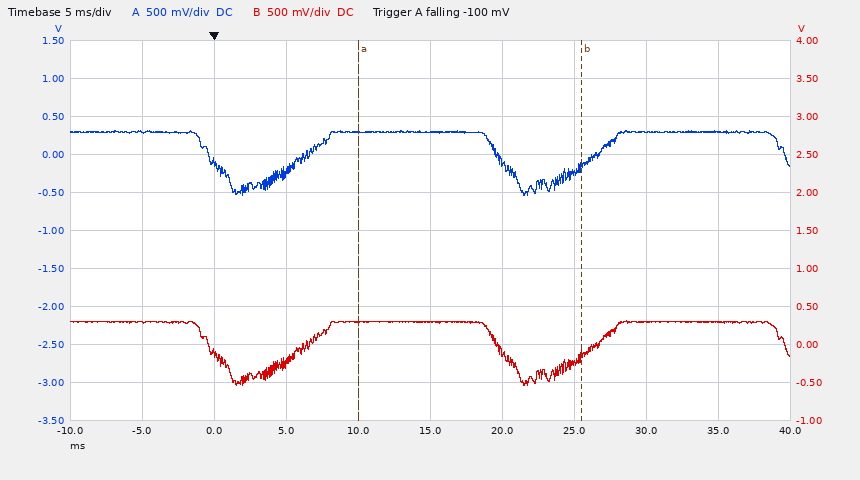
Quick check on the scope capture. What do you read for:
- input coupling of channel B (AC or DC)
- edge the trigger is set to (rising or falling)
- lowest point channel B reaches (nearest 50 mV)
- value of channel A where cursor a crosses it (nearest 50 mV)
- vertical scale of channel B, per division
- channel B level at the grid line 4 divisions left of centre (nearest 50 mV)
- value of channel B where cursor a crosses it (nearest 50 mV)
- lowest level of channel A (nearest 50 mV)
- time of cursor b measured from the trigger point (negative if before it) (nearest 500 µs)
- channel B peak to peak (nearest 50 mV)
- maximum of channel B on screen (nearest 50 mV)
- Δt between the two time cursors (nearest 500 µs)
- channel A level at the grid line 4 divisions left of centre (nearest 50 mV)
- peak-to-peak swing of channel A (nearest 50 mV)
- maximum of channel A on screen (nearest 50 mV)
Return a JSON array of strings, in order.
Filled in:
["DC", "falling", "-550 mV", "300 mV", "500 mV", "300 mV", "300 mV", "-550 mV", "+25.5 ms", "850 mV", "300 mV", "15.5 ms", "300 mV", "850 mV", "300 mV"]
